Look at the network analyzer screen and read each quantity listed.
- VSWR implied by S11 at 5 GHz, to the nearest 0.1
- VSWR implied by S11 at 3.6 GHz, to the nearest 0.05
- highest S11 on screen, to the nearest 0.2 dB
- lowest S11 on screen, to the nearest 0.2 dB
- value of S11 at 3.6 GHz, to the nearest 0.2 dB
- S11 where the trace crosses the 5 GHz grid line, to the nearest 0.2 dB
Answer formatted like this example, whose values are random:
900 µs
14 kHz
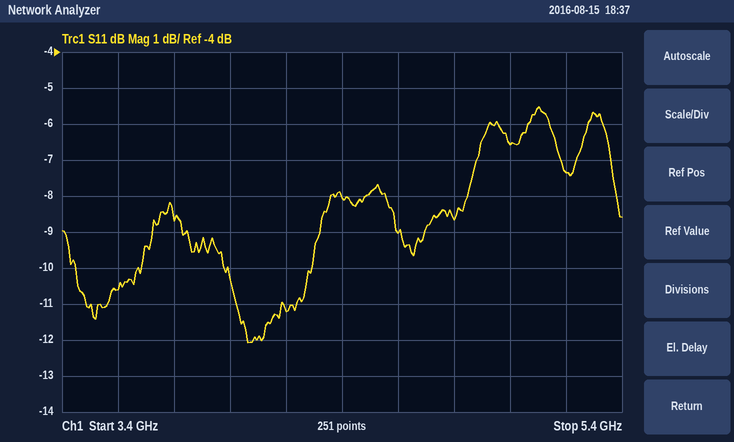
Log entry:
2.8
1.85
-5.6 dB
-12.0 dB
-10.6 dB
-6.6 dB
